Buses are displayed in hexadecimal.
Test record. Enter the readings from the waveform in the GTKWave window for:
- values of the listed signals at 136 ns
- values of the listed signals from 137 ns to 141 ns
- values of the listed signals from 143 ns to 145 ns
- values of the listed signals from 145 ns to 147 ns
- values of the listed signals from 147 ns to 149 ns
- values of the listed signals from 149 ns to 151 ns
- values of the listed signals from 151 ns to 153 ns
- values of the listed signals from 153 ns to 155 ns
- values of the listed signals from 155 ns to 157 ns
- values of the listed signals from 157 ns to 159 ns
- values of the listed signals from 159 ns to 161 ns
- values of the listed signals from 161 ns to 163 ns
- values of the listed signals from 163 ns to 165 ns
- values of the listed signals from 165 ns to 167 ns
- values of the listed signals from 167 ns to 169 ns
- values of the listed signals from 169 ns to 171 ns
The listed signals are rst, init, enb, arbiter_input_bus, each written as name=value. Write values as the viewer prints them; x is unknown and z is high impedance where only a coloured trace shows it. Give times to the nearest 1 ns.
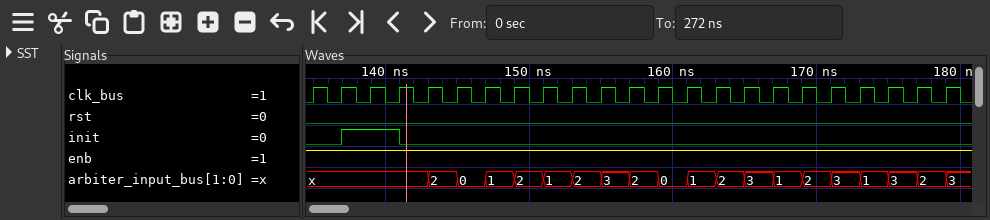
rst=0, init=0, enb=1, arbiter_input_bus=x
rst=0, init=1, enb=1, arbiter_input_bus=x
rst=0, init=0, enb=1, arbiter_input_bus=2
rst=0, init=0, enb=1, arbiter_input_bus=0
rst=0, init=0, enb=1, arbiter_input_bus=1
rst=0, init=0, enb=1, arbiter_input_bus=2
rst=0, init=0, enb=1, arbiter_input_bus=1
rst=0, init=0, enb=1, arbiter_input_bus=2
rst=0, init=0, enb=1, arbiter_input_bus=3
rst=0, init=0, enb=1, arbiter_input_bus=2
rst=0, init=0, enb=1, arbiter_input_bus=0
rst=0, init=0, enb=1, arbiter_input_bus=1
rst=0, init=0, enb=1, arbiter_input_bus=2
rst=0, init=0, enb=1, arbiter_input_bus=3
rst=0, init=0, enb=1, arbiter_input_bus=1
rst=0, init=0, enb=1, arbiter_input_bus=2
